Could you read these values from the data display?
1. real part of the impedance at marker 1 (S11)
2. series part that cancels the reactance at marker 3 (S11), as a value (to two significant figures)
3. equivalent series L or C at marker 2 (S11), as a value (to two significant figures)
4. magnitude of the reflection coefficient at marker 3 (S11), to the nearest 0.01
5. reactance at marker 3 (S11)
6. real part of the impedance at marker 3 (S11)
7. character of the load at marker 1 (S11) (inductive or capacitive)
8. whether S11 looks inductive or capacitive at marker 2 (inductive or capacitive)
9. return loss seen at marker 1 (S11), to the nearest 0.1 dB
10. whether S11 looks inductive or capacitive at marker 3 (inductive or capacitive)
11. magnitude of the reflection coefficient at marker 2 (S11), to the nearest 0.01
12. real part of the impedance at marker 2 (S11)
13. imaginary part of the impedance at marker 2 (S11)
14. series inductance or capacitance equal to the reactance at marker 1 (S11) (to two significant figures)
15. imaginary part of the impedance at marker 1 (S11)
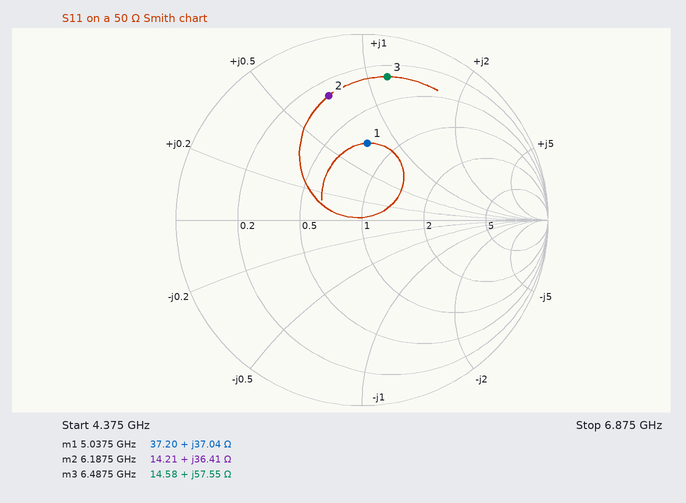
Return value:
37.20 Ω
430 fF
940 pH
0.78
+57.55 Ω
14.58 Ω
inductive
inductive
7.7 dB
inductive
0.69
14.21 Ω
+36.41 Ω
1.2 nH
+37.04 Ω
